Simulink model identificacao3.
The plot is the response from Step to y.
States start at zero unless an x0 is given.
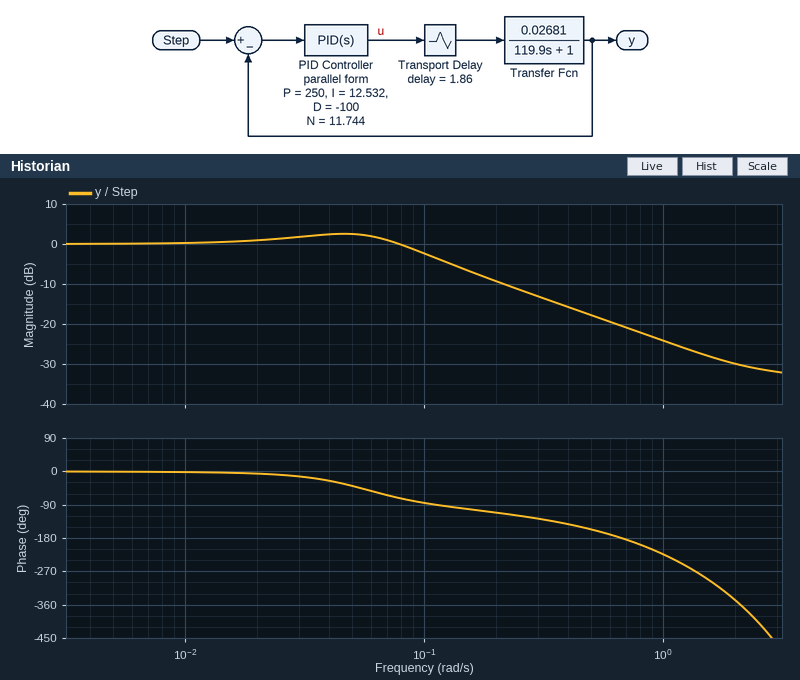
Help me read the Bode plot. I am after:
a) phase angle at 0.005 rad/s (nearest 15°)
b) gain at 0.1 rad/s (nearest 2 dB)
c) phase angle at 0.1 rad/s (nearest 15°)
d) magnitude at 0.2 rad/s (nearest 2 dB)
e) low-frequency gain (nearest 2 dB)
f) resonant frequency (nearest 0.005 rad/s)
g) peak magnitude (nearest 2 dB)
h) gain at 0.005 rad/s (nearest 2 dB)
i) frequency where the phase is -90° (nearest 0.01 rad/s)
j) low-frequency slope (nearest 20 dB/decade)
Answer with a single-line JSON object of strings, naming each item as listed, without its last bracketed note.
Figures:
{"phase angle at 0.005 rad/s": "0°", "gain at 0.1 rad/s": "-2 dB", "phase angle at 0.1 rad/s": "-90°", "magnitude at 0.2 rad/s": "-10 dB", "low-frequency gain": "0 dB", "resonant frequency": "0.045 rad/s", "peak magnitude": "2 dB", "gain at 0.005 rad/s": "0 dB", "frequency where the phase is -90°": "0.11 rad/s", "low-frequency slope": "0 dB/decade"}
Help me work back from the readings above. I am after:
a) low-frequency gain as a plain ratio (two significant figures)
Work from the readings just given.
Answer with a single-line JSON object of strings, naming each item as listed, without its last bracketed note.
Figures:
{"low-frequency gain as a plain ratio": "1.0"}
